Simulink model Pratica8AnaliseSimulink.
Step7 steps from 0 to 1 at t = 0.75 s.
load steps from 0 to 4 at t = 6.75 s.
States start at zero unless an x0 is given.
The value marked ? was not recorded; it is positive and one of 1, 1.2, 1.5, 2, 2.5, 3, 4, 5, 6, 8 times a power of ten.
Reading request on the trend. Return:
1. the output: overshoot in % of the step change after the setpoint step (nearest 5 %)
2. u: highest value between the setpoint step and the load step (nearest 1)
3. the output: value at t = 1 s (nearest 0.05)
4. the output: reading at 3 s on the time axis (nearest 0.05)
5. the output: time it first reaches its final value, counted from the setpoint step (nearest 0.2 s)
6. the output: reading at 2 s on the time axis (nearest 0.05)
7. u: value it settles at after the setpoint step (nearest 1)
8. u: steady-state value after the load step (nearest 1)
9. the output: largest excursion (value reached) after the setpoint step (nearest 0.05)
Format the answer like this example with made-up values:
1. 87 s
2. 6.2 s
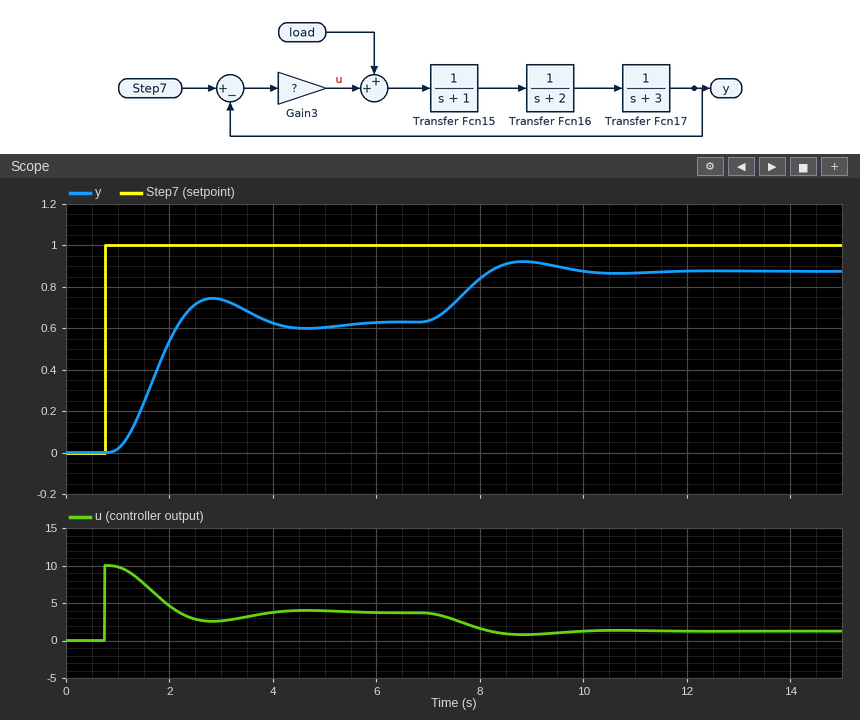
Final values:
1. 20 %
2. 10
3. 0.00
4. 0.75
5. 1.4 s
6. 0.55
7. 4
8. 1
9. 0.75
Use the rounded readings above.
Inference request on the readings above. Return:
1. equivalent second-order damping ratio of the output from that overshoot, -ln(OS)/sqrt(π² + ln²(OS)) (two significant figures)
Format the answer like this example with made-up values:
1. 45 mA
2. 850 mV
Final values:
1. 0.46
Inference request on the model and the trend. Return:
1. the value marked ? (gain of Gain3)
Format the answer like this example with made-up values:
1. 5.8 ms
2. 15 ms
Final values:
1. 10
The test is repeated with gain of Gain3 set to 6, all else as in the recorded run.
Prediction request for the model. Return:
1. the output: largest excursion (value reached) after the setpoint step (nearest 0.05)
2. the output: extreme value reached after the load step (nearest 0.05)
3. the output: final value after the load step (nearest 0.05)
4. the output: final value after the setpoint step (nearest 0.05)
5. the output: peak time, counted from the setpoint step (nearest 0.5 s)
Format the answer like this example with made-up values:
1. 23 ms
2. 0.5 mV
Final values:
1. 0.55
2. 0.85
3. 0.85
4. 0.50
5. 2.5 s
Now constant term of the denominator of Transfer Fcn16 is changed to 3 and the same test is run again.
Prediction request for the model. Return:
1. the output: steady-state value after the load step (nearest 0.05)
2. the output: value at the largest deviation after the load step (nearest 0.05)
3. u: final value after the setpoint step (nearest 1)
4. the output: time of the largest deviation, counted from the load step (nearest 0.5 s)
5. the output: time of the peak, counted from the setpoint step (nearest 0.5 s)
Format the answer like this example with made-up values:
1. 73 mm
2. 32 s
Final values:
1. 0.75
2. 0.75
3. 5
4. 2.0 s
5. 2.0 s
